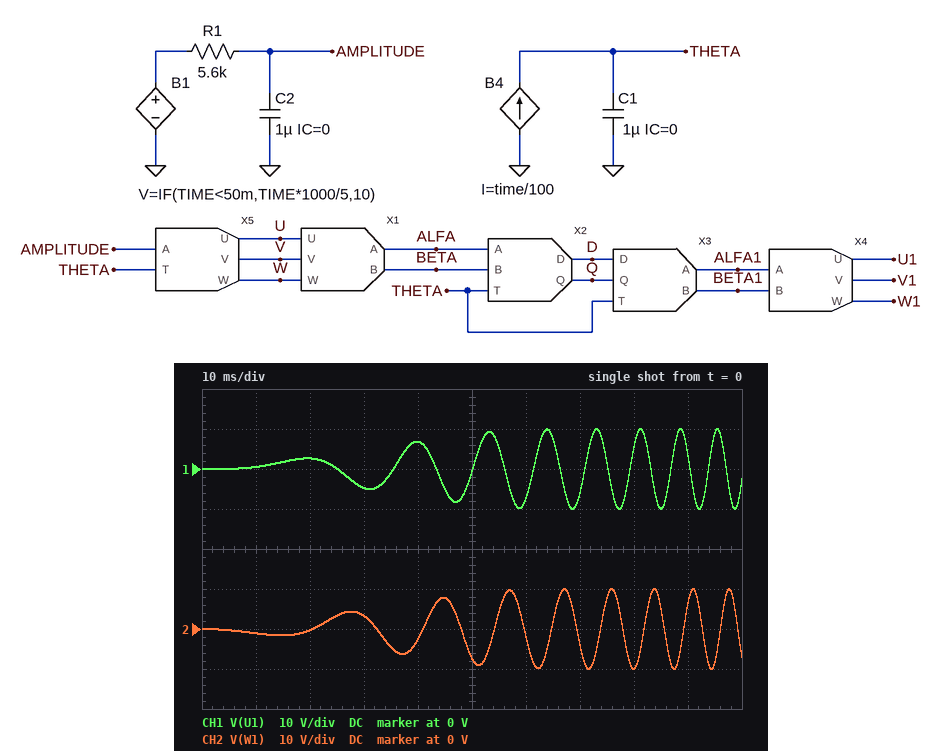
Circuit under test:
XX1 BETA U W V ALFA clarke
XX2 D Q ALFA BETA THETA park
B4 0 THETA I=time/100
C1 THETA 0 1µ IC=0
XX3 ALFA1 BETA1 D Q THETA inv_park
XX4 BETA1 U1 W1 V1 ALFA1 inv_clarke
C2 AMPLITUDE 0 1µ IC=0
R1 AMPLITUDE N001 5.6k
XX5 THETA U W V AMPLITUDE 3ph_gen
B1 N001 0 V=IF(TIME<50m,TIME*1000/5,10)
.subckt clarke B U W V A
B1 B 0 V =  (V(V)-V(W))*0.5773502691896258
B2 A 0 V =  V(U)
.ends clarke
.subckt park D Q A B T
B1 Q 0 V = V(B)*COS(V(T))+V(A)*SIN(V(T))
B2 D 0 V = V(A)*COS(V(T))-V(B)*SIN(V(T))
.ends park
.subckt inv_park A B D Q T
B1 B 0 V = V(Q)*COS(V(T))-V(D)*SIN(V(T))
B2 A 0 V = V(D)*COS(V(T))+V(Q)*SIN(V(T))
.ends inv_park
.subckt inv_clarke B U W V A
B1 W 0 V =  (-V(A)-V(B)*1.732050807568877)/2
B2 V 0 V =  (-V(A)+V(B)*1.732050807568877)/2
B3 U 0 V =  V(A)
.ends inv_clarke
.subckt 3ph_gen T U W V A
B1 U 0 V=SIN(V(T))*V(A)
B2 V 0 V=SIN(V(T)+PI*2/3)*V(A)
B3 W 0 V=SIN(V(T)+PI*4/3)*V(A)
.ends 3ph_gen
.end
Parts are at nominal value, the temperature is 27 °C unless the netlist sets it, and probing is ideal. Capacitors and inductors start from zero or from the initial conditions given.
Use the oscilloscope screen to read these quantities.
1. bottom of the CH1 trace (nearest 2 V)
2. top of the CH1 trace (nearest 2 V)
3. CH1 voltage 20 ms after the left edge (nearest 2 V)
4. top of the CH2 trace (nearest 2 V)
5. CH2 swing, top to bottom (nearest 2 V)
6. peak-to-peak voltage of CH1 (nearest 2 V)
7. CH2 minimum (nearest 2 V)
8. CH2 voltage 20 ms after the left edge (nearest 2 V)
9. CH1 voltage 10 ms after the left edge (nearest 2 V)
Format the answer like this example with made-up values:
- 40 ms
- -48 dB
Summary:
- -10 V
- 10 V
- 2 V
- 10 V
- 20 V
- 20 V
- -10 V
- 0 V
- 0 V
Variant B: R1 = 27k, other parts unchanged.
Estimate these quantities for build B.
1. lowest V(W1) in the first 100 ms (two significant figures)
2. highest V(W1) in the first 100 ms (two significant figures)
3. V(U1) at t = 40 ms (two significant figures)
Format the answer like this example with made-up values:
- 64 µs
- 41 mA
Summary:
- -9.1 V
- 9.2 V
- 3.8 V
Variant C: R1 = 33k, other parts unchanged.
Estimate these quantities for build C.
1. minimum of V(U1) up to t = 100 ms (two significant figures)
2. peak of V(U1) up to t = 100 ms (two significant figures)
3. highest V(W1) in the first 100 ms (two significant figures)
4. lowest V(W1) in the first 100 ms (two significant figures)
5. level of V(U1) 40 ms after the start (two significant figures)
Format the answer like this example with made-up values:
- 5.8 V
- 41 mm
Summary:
- -8.8 V
- 8.7 V
- 8.8 V
- -8.7 V
- 3.3 V
